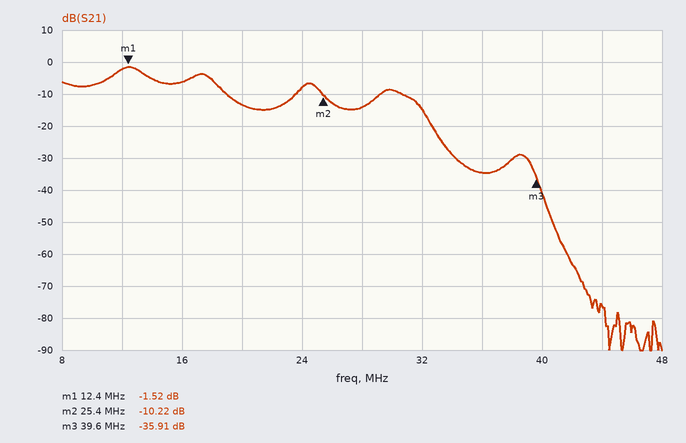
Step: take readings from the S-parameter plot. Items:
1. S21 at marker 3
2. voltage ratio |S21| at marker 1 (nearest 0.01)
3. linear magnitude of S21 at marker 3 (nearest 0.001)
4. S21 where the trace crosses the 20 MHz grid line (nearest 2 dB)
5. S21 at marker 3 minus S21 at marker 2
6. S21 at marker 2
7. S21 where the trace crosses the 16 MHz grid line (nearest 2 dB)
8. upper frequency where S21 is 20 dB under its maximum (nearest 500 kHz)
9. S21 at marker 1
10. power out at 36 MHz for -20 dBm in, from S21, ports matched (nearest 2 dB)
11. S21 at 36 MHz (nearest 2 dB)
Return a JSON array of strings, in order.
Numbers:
["-35.91 dB", "0.84", "0.016", "-14 dB", "-25.69 dB", "-10.22 dB", "-6 dB", "33.0 MHz", "-1.52 dB", "-54 dBm", "-34 dB"]
